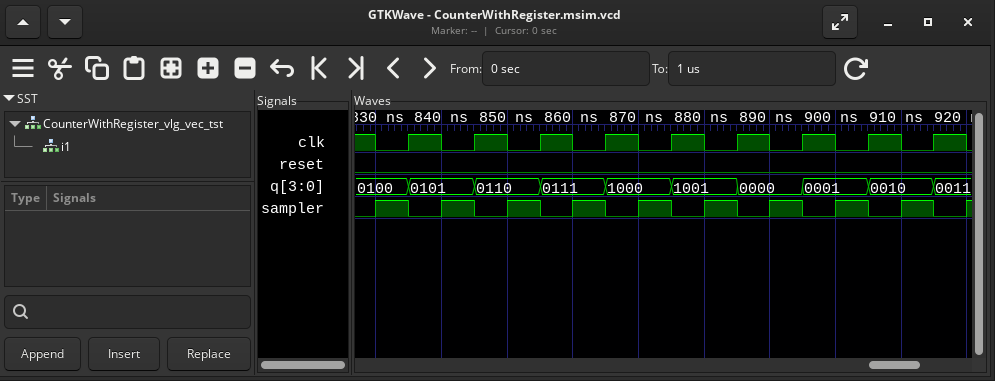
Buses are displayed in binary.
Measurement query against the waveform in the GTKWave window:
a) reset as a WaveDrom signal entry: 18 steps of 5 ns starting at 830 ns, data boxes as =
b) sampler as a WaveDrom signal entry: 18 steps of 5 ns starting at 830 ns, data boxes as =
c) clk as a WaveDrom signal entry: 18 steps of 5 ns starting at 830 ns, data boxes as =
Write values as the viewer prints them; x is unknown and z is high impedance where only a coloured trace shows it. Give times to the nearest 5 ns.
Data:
{name: 'reset', wave: '0.................'}
{name: 'sampler', wave: '101010101010101010'}
{name: 'clk', wave: '010101010101010101'}
